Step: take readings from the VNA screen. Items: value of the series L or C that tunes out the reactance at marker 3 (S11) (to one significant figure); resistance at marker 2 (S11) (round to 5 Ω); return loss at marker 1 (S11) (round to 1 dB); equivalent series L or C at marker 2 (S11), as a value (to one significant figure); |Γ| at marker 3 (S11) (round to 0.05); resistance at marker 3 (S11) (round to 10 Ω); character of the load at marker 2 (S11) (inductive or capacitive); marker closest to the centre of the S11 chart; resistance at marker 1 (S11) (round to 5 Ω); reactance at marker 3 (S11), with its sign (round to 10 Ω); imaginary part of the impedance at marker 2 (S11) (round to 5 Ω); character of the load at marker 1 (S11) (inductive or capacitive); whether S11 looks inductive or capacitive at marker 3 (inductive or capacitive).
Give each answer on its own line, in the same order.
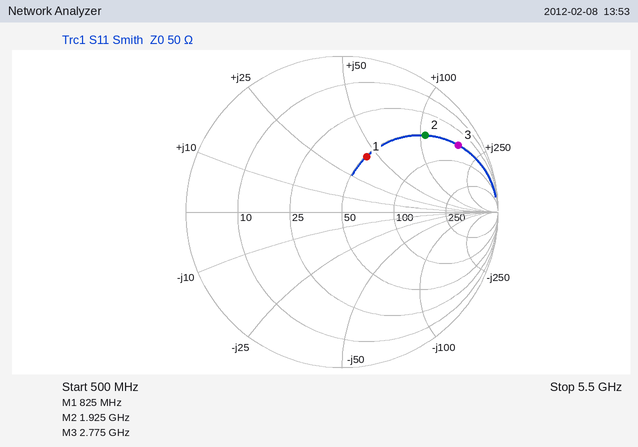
300 fF
50 Ω
8 dB
9 nH
0.85
50 Ω
inductive
marker 1
50 Ω
+170 Ω
+105 Ω
inductive
inductive
